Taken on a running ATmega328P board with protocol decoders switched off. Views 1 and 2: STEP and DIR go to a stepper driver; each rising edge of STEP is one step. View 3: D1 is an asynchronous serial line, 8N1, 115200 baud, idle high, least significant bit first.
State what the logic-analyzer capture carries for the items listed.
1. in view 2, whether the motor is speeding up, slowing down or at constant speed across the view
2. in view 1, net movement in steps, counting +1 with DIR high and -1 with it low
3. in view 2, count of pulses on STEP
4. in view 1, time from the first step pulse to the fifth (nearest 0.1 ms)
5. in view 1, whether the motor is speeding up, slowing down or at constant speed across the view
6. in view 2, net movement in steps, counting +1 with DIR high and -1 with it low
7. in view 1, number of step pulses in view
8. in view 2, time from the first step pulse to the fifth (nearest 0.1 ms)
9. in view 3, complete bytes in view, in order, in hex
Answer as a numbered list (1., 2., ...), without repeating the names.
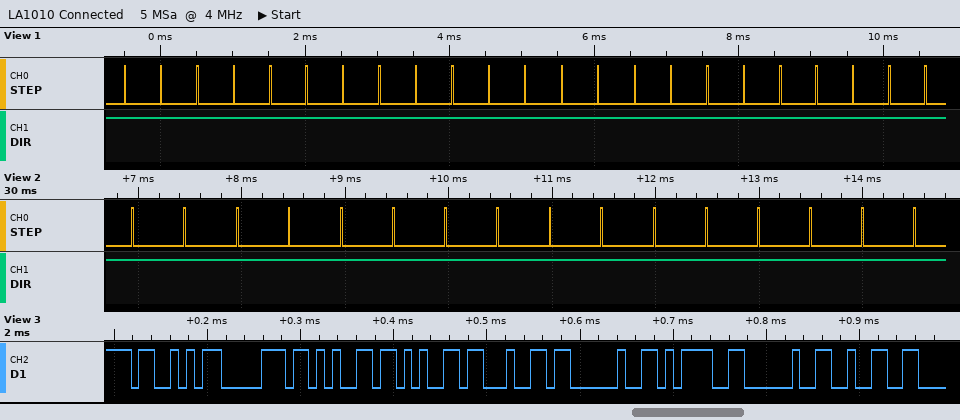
1. constant speed
2. +23
3. 16
4. 2.0 ms
5. constant speed
6. +16
7. 23
8. 2.0 ms
9. 53 70 65 65 64 20 3D 20 32
